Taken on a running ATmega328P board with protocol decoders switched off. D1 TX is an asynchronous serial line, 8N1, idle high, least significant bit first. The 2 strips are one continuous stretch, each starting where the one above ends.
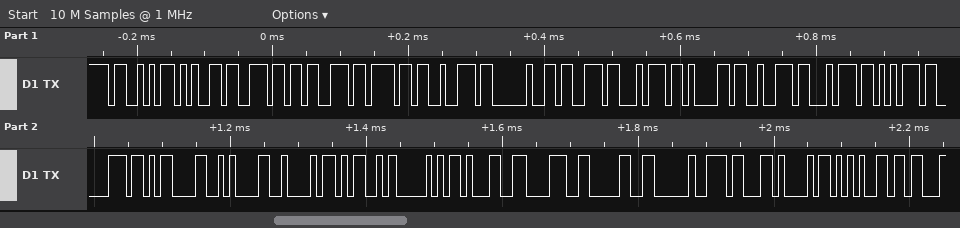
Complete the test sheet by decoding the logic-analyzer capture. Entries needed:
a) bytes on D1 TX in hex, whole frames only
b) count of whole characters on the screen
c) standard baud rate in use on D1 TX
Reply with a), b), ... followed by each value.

a) 0x53 0x65 0x6E 0x73 0x6F 0x72 0x20 0x73 0x74 0x61 0x72 0x74 0x75 0x70 0x0D 0x0A 0x42 0x4D 0x50 0x31 0x38 0x30 0x20 0x63 0x68 0x65
b) 26
c) 115200 baud
